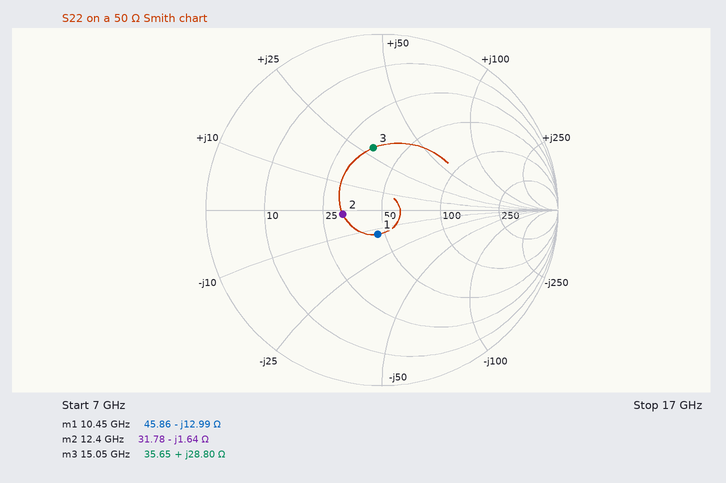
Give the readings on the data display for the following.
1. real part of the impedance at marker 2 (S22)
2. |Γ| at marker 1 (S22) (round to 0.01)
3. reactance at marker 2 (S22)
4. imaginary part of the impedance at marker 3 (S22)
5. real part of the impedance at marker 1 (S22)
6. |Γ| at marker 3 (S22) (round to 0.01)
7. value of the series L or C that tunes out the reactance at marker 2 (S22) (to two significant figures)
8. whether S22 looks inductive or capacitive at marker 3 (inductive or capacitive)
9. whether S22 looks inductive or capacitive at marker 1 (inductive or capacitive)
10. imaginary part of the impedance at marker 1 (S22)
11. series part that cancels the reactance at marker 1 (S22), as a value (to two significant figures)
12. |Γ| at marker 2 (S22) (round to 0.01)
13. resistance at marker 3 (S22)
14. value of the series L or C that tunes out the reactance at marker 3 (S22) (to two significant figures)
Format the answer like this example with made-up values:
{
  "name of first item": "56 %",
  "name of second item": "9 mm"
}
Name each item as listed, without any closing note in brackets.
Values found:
{
  "real part of the impedance at marker 2": "31.78 Ω",
  "|Γ| at marker 1 (S22)": "0.14",
  "reactance at marker 2": "-1.64 Ω",
  "imaginary part of the impedance at marker 3": "+28.80 Ω",
  "real part of the impedance at marker 1": "45.86 Ω",
  "|Γ| at marker 3 (S22)": "0.36",
  "value of the series L or C that tunes out the reactance at marker 2 (S22)": "21 pH",
  "whether S22 looks inductive or capacitive at marker 3": "inductive",
  "whether S22 looks inductive or capacitive at marker 1": "capacitive",
  "imaginary part of the impedance at marker 1": "-12.99 Ω",
  "series part that cancels the reactance at marker 1 (S22), as a value": "200 pH",
  "|Γ| at marker 2 (S22)": "0.22",
  "resistance at marker 3": "35.65 Ω",
  "value of the series L or C that tunes out the reactance at marker 3 (S22)": "370 fF"
}
